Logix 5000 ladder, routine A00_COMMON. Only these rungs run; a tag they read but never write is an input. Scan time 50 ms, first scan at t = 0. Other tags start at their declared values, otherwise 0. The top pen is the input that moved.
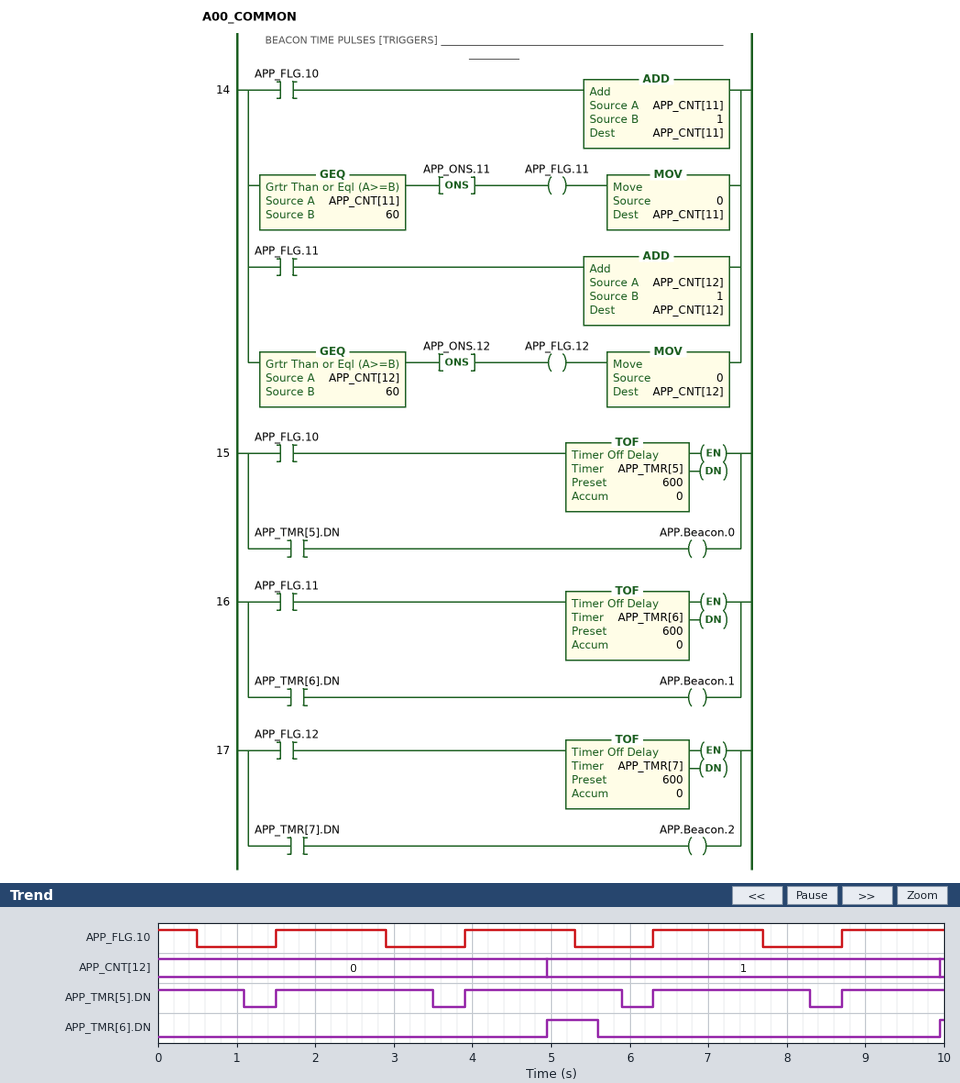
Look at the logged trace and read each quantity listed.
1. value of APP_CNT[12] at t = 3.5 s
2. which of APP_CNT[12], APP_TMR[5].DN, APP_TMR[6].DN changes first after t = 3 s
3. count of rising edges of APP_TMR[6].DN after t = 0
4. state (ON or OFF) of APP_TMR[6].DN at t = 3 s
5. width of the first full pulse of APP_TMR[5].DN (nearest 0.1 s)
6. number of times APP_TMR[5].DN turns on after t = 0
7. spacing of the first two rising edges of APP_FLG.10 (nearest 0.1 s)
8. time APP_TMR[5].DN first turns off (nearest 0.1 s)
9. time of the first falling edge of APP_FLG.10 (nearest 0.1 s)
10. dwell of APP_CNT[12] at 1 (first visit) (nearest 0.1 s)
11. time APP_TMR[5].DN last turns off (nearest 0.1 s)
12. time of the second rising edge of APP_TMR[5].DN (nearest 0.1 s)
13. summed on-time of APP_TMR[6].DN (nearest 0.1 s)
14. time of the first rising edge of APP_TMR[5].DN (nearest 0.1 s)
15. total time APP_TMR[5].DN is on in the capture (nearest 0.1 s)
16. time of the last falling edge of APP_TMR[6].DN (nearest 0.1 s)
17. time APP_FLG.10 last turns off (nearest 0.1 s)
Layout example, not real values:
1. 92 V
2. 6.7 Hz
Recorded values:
1. 0
2. APP_TMR[5].DN
3. 2
4. OFF
5. 2.0 s
6. 4
7. 2.4 s
8. 1.1 s
9. 0.5 s
10. 5.0 s
11. 8.3 s
12. 3.9 s
13. 0.7 s
14. 1.5 s
15. 8.4 s
16. 5.6 s
17. 7.7 s
